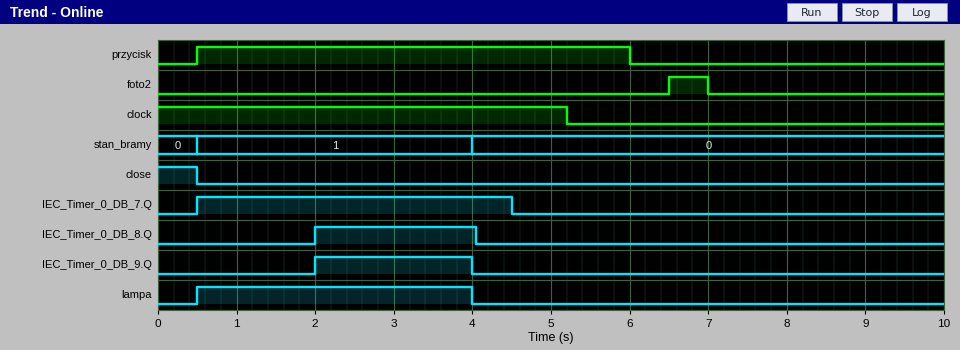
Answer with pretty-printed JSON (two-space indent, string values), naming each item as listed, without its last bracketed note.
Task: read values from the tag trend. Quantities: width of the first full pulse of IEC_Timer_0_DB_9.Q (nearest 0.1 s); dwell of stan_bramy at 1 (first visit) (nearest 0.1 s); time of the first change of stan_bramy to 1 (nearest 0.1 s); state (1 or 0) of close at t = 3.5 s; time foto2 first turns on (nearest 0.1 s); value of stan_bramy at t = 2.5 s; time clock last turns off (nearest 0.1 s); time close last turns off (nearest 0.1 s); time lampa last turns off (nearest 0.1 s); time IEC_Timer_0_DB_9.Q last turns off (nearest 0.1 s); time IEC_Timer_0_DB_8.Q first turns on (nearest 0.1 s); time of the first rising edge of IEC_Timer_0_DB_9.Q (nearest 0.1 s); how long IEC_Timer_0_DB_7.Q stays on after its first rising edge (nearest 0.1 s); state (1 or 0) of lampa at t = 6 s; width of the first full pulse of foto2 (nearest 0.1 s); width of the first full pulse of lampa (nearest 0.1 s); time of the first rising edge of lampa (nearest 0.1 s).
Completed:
{
  "width of the first full pulse of IEC_Timer_0_DB_9.Q": "2.0 s",
  "dwell of stan_bramy at 1 (first visit)": "3.5 s",
  "time of the first change of stan_bramy to 1": "0.5 s",
  "state (1 or 0) of close at t = 3.5 s": "0",
  "time foto2 first turns on": "6.5 s",
  "value of stan_bramy at t = 2.5 s": "1",
  "time clock last turns off": "5.2 s",
  "time close last turns off": "0.5 s",
  "time lampa last turns off": "4.0 s",
  "time IEC_Timer_0_DB_9.Q last turns off": "4.0 s",
  "time IEC_Timer_0_DB_8.Q first turns on": "2.0 s",
  "time of the first rising edge of IEC_Timer_0_DB_9.Q": "2.0 s",
  "how long IEC_Timer_0_DB_7.Q stays on after its first rising edge": "4.0 s",
  "state (1 or 0) of lampa at t = 6 s": "0",
  "width of the first full pulse of foto2": "0.5 s",
  "width of the first full pulse of lampa": "3.5 s",
  "time of the first rising edge of lampa": "0.5 s"
}
